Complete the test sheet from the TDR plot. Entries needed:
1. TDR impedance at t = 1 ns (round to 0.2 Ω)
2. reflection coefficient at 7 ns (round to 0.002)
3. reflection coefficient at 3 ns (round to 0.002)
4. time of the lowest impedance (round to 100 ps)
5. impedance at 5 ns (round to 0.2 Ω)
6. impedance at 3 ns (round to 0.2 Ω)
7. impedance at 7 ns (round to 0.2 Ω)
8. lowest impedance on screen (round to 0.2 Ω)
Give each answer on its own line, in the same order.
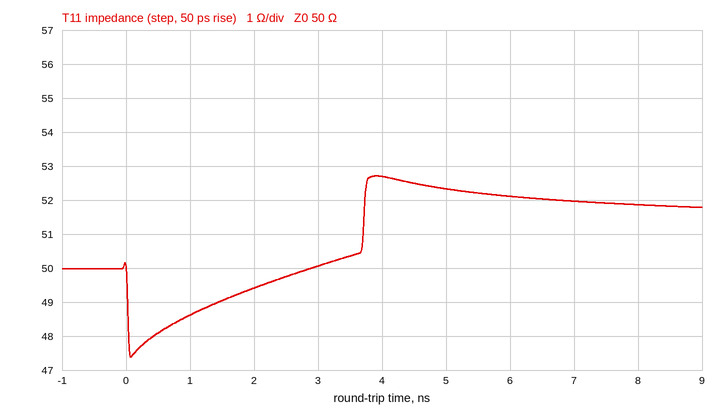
48.6 Ω
+0.020
0.000
100 ps
52.4 Ω
50.0 Ω
52.0 Ω
47.4 Ω
